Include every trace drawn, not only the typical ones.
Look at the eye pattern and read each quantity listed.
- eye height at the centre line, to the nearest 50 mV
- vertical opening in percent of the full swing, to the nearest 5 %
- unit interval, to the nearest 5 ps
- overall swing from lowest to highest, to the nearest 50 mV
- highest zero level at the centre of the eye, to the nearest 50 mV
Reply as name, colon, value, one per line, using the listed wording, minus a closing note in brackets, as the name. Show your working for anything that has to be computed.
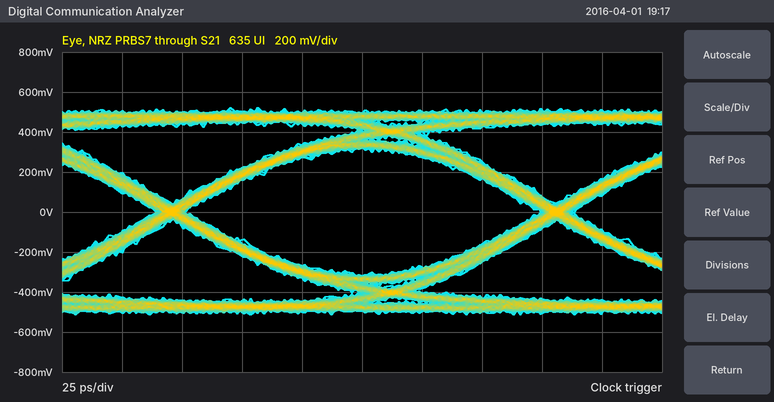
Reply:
eye height at the centre line, to the nearest 50 mV: 650 mV
vertical opening in percent of the full swing, to the nearest 5 %: 650 mV / 1.05 V ≈ 61.9 %, so 60 % to the nearest 5 %
unit interval, to the nearest 5 ps: 160 ps
overall swing from lowest to highest, to the nearest 50 mV: 1.05 V
highest zero level at the centre of the eye, to the nearest 50 mV: -300 mV
